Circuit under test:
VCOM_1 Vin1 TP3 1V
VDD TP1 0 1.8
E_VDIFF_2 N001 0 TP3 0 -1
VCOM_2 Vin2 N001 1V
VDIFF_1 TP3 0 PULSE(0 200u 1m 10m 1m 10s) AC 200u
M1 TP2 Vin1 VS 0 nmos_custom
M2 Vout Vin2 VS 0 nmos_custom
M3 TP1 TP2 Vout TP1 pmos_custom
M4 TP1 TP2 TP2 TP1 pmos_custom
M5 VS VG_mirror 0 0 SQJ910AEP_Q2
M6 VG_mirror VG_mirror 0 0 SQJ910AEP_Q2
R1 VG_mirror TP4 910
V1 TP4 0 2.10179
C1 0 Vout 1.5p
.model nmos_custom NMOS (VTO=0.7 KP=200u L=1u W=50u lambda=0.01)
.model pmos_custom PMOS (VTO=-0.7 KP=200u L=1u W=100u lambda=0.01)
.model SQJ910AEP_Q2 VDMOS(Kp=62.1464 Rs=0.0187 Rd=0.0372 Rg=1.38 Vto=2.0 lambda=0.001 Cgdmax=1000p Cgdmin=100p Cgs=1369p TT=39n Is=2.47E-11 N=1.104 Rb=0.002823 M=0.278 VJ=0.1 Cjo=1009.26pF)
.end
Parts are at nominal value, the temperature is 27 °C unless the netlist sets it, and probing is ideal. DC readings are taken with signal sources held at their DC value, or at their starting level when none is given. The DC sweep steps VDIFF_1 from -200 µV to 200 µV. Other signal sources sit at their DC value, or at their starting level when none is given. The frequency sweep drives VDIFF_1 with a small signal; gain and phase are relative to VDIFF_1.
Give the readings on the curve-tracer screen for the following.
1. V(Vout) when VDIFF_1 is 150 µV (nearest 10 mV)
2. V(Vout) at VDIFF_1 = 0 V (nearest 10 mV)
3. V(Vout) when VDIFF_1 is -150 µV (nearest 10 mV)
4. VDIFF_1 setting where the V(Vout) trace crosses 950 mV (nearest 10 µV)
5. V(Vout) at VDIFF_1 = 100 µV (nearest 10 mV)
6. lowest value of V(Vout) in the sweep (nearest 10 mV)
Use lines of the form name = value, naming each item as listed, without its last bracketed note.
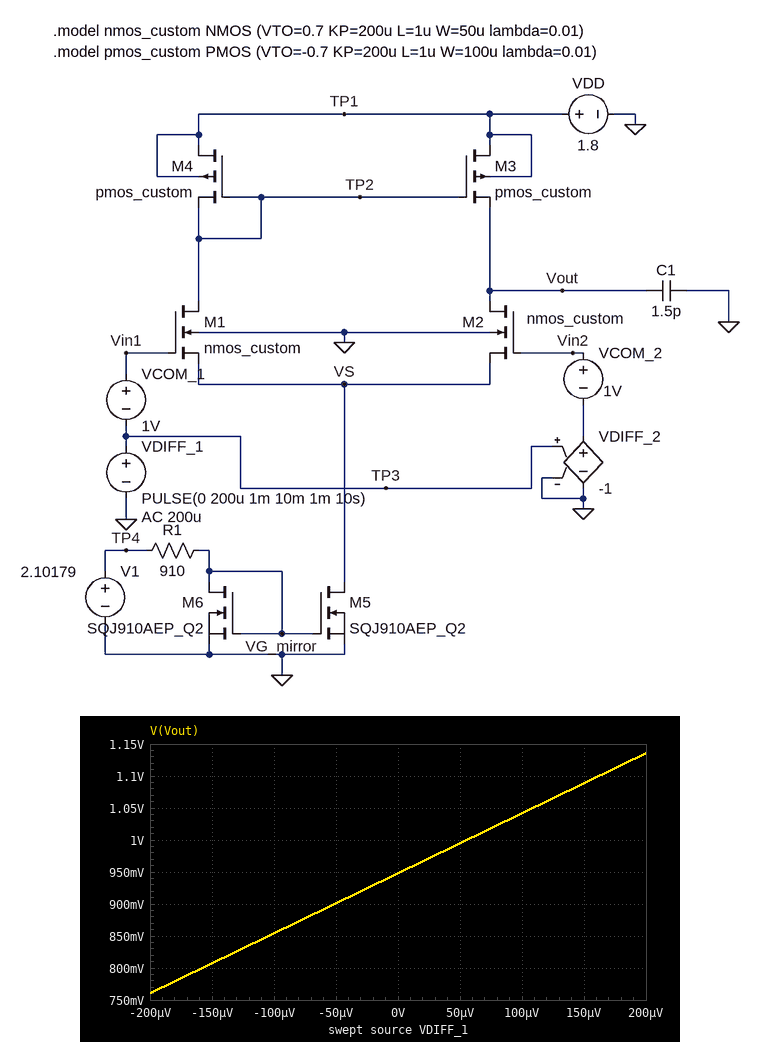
V(Vout) when VDIFF_1 is 150 µV = 1.09 V
V(Vout) at VDIFF_1 = 0 V = 950 mV
V(Vout) when VDIFF_1 is -150 µV = 810 mV
VDIFF_1 setting where the V(Vout) trace crosses 950 mV = 0 V
V(Vout) at VDIFF_1 = 100 µV = 1.04 V
lowest value of V(Vout) in the sweep = 760 mV
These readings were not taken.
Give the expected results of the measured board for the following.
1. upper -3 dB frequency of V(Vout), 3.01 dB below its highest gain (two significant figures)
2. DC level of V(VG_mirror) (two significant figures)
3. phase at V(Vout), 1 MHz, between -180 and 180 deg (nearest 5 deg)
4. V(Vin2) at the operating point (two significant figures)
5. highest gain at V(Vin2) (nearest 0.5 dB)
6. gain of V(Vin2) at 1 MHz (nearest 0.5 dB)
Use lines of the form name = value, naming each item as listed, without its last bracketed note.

upper -3 dB frequency of V(Vout), 3.01 dB below its highest gain = 490 kHz
DC level of V(VG_mirror) = 1.7 V
phase at V(Vout), 1 MHz, between -180 and 180 deg = -65 deg
V(Vin2) at the operating point = 1.0 V
highest gain at V(Vin2) = 0 dB
gain of V(Vin2) at 1 MHz = 0 dB
